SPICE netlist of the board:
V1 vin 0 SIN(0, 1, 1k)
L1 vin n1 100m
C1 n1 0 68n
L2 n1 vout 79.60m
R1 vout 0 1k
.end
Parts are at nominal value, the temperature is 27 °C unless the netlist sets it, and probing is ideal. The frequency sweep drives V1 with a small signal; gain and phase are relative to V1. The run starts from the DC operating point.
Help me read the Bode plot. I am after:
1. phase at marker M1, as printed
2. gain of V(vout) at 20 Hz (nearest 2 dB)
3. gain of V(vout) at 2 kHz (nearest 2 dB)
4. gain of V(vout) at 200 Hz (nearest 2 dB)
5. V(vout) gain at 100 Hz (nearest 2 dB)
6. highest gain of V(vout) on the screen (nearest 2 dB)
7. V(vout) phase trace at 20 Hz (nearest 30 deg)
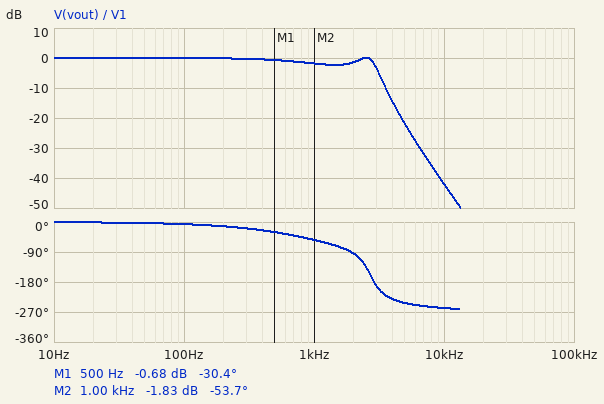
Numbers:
-30.4 deg
0 dB
-2 dB
0 dB
0 dB
0 dB
0 deg
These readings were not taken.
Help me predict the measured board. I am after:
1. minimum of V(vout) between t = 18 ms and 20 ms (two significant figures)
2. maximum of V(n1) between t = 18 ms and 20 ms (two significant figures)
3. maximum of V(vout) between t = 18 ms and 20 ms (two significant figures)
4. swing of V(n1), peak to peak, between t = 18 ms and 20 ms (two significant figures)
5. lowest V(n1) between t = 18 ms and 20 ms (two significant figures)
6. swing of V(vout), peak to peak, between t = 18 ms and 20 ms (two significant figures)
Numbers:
-810 mV
910 mV
810 mV
1.8 V
-910 mV
1.6 V
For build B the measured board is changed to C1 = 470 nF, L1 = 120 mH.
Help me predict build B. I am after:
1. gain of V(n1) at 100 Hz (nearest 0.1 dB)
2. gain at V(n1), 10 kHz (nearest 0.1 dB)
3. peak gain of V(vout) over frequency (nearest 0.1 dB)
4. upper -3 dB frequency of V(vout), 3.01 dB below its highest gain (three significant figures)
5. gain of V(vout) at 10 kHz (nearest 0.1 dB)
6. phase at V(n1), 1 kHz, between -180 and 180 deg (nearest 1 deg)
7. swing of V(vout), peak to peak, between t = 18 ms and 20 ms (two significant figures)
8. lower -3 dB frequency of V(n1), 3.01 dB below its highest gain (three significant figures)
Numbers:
0.1 dB
-46.9 dB
6.0 dB
847 Hz
-61.0 dB
-147 deg
1.6 V
473 Hz
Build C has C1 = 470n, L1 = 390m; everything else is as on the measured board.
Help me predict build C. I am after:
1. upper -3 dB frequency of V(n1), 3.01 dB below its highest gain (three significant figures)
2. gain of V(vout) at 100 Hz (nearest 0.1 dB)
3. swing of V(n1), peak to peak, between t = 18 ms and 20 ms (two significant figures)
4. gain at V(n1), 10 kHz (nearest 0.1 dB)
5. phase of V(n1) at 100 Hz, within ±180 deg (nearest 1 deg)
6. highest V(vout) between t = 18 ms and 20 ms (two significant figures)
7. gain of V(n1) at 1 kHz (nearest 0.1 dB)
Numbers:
486 Hz
0.2 dB
360 mV
-57.1 dB
-15 deg
160 mV
-15.0 dB
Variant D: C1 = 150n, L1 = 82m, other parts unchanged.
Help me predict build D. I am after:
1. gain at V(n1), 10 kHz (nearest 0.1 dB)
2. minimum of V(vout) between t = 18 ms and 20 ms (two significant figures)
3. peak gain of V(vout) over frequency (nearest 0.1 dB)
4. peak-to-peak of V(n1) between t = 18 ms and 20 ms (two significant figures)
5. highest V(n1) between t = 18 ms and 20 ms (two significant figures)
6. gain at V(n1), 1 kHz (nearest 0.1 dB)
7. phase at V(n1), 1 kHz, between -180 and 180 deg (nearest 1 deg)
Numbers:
-33.4 dB
-1.1 V
3.5 dB
2.4 V
1.2 V
1.6 dB
-30 deg
